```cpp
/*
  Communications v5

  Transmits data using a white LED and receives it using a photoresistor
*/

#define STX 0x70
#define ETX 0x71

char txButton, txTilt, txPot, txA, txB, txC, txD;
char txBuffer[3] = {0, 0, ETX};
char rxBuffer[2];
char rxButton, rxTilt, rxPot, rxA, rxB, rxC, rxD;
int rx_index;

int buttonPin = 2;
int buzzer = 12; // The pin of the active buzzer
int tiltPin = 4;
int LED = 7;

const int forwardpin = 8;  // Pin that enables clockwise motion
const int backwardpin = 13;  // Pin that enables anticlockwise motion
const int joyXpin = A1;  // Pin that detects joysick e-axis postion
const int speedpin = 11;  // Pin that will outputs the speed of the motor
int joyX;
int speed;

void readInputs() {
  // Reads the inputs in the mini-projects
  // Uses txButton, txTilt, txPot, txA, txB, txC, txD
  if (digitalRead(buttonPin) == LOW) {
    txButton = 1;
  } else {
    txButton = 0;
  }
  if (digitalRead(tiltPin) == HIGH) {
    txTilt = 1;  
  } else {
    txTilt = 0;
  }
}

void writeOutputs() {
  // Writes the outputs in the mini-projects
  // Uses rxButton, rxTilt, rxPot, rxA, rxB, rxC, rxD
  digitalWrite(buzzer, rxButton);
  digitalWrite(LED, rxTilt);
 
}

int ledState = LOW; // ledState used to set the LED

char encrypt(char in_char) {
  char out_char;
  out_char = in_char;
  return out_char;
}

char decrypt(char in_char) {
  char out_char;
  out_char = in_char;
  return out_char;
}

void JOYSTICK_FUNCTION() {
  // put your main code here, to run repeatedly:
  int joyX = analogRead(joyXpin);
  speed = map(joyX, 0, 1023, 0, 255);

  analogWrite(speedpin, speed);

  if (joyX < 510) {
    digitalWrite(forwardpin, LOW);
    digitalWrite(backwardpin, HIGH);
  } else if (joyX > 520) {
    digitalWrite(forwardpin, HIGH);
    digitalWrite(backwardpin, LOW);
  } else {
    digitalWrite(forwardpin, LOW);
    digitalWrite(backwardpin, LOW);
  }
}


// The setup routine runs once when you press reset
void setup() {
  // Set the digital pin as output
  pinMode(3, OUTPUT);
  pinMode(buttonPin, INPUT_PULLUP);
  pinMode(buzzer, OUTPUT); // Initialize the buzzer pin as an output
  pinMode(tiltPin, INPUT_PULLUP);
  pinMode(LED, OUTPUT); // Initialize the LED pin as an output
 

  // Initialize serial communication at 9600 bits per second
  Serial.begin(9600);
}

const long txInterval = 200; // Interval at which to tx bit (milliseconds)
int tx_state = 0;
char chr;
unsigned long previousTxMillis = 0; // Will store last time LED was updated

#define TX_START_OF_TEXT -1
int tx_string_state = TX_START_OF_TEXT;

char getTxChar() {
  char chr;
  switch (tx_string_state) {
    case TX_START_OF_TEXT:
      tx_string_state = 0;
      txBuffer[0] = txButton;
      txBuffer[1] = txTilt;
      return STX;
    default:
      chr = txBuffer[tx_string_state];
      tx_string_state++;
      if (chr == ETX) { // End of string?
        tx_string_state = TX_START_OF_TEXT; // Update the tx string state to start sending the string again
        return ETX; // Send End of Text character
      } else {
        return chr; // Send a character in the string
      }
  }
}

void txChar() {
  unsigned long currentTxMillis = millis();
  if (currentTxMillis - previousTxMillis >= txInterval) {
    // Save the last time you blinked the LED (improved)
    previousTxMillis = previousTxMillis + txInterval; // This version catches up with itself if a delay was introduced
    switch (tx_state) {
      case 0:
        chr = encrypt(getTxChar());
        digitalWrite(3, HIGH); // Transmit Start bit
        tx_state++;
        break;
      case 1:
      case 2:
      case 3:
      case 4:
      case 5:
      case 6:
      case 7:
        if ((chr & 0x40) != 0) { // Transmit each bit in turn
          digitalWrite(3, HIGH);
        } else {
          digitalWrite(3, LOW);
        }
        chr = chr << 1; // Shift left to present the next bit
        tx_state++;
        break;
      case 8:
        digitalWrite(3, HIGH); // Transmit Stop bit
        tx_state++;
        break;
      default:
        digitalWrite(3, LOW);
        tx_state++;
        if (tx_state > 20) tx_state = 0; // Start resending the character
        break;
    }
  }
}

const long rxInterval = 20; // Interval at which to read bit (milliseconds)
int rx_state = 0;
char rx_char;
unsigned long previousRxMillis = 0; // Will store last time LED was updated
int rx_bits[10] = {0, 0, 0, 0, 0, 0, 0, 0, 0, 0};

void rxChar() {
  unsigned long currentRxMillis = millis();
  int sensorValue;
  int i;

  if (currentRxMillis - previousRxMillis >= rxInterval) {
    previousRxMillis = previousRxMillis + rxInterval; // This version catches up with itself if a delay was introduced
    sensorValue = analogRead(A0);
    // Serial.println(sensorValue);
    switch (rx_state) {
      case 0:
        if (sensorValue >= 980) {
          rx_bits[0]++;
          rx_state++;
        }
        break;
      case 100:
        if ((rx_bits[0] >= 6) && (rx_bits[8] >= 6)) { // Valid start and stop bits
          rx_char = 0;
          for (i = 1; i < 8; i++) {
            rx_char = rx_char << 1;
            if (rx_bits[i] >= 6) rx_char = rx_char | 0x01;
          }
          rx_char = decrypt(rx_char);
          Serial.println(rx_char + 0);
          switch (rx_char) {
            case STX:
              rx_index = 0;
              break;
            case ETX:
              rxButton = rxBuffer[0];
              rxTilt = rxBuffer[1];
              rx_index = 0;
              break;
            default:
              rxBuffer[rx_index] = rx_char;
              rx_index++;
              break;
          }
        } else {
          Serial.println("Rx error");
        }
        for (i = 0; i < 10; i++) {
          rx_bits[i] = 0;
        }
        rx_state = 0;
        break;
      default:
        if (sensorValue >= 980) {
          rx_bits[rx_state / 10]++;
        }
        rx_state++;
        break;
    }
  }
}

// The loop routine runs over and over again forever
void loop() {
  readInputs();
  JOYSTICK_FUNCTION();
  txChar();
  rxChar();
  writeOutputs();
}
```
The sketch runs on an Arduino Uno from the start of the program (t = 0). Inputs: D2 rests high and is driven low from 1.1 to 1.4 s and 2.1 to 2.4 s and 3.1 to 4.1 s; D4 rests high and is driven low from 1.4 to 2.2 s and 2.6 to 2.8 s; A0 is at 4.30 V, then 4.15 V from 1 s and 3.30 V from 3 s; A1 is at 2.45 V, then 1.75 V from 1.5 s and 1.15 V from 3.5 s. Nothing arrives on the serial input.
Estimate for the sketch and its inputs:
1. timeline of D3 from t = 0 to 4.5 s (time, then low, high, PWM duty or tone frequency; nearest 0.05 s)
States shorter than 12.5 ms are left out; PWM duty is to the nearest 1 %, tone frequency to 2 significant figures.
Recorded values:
0 s low; 0.2 s high; 1 s low; 1.8 s high; 2 s low; 4.4 s high
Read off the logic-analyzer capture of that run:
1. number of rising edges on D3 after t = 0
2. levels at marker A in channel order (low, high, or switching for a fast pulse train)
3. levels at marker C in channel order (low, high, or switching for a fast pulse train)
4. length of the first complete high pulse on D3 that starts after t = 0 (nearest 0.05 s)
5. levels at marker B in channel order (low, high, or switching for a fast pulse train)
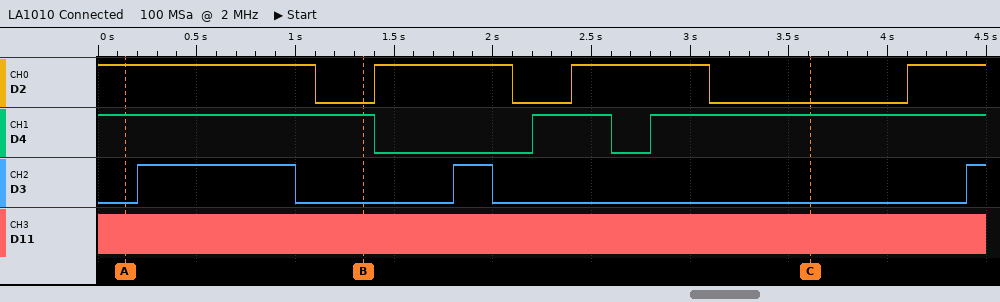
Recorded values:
3
D2 high, D4 high, D3 low, D11 switching
D2 low, D4 high, D3 low, D11 switching
0.80 s
D2 low, D4 high, D3 low, D11 switching
